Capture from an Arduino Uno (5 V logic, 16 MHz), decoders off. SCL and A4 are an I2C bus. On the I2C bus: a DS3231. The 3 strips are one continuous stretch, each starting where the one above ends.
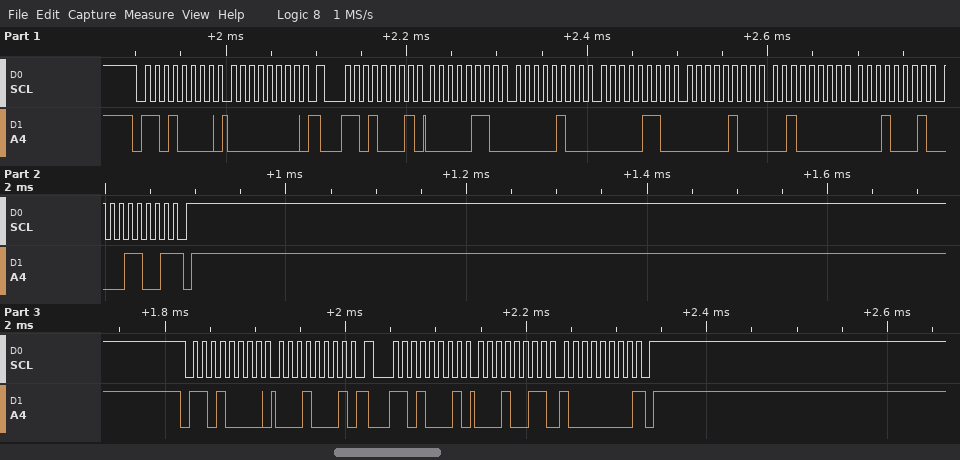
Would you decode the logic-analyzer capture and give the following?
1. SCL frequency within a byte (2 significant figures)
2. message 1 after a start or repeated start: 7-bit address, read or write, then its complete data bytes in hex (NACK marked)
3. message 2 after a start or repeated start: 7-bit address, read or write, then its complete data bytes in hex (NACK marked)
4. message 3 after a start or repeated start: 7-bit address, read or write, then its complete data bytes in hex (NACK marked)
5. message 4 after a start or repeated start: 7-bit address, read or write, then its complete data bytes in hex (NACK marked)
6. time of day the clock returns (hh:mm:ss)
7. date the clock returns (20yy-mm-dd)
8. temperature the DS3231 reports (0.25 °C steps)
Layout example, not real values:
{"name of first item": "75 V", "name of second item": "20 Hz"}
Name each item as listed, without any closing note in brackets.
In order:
{"SCL frequency within a byte": "100 kHz", "message 1 after a start or repeated start: 7-bit address, read or write, then its complete data bytes in hex": "0x68 write: 00", "message 2 after a start or repeated start: 7-bit address, read or write, then its complete data bytes in hex": "0x68 read: 06 04 06 04 20 11 19 NACK", "message 3 after a start or repeated start: 7-bit address, read or write, then its complete data bytes in hex": "0x68 write: 11", "message 4 after a start or repeated start: 7-bit address, read or write, then its complete data bytes in hex": "0x68 read: 13 80 NACK", "time of day the clock returns": "06:04:06", "date the clock returns": "2019-11-20", "temperature the DS3231 reports": "19.50 °C"}
